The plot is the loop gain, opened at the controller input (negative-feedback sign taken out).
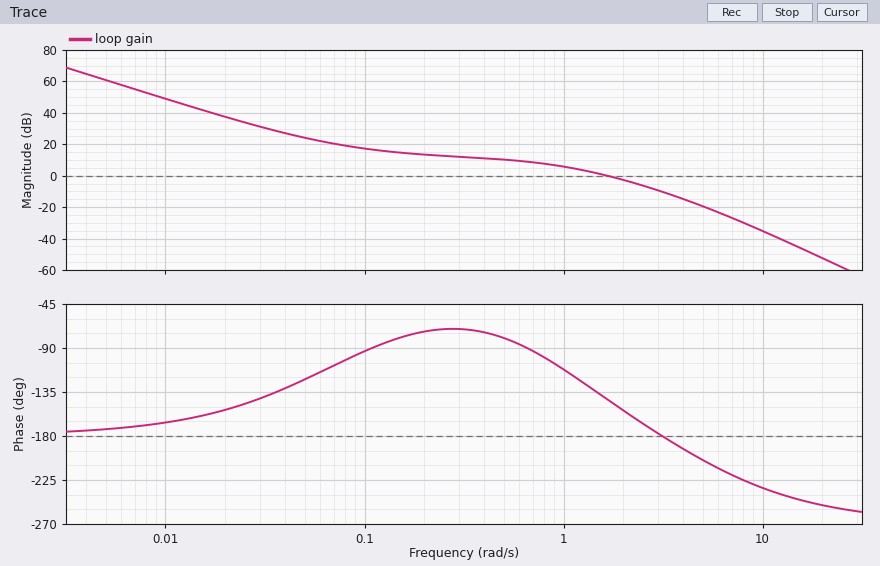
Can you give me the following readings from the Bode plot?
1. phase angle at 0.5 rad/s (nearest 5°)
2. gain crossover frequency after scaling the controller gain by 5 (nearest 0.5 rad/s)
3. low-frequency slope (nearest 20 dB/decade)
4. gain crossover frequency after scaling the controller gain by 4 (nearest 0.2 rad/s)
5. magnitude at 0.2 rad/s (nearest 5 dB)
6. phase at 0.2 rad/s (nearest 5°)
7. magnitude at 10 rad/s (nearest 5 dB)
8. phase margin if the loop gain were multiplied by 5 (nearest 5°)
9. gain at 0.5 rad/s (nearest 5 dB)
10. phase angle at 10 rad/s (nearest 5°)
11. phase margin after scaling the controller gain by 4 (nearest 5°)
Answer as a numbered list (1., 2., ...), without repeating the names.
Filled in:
1. -80°
2. 4.0 rad/s
3. -40 dB/decade
4. 3.4 rad/s
5. 15 dB
6. -75°
7. -35 dB
8. -10°
9. 10 dB
10. -235°
11. -5°
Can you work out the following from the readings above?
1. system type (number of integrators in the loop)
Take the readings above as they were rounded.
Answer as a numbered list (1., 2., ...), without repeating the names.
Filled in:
1. 2
